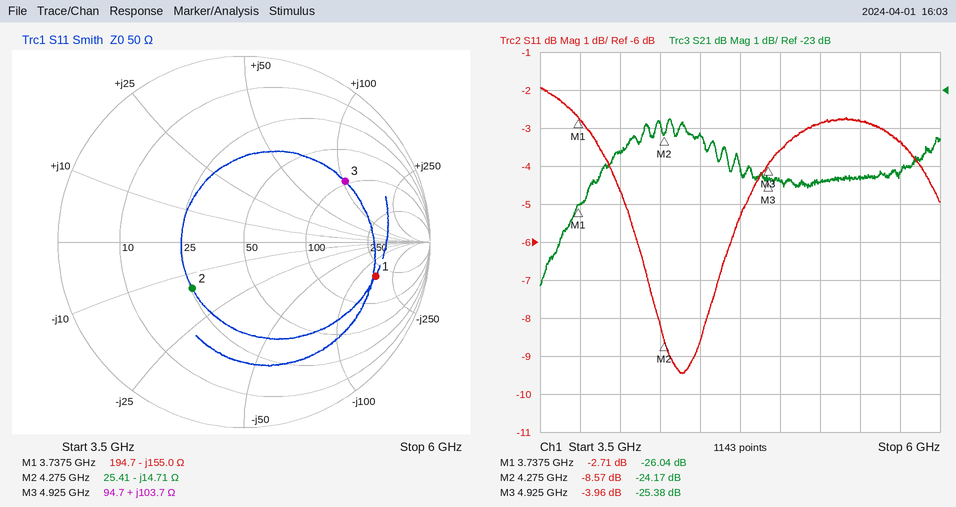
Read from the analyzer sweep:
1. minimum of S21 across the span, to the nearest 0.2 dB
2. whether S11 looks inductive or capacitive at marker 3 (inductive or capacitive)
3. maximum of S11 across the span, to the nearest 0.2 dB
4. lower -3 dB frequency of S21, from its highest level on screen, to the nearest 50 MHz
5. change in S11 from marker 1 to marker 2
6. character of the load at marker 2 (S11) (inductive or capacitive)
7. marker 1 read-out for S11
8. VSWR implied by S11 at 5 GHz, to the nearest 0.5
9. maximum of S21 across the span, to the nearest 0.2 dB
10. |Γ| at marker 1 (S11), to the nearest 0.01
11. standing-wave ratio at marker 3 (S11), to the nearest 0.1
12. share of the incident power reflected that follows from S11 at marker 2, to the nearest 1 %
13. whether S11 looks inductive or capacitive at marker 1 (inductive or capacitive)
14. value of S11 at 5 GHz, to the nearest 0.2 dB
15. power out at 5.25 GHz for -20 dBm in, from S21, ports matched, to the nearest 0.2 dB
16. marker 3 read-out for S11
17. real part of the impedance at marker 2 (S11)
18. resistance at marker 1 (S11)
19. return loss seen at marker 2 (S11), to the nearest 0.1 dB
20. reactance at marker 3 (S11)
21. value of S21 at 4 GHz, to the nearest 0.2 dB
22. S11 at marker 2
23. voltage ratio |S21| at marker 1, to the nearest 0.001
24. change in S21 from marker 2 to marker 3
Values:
-28.2 dB
inductive
-2.0 dB
3.65 GHz
-5.86 dB
capacitive
-2.71 dB
5.0
-23.8 dB
0.73
4.5
14 %
capacitive
-3.6 dB
-45.4 dBm
-3.96 dB
25.41 Ω
194.7 Ω
8.6 dB
+103.7 Ω
-24.6 dB
-8.57 dB
0.050
-1.21 dB
